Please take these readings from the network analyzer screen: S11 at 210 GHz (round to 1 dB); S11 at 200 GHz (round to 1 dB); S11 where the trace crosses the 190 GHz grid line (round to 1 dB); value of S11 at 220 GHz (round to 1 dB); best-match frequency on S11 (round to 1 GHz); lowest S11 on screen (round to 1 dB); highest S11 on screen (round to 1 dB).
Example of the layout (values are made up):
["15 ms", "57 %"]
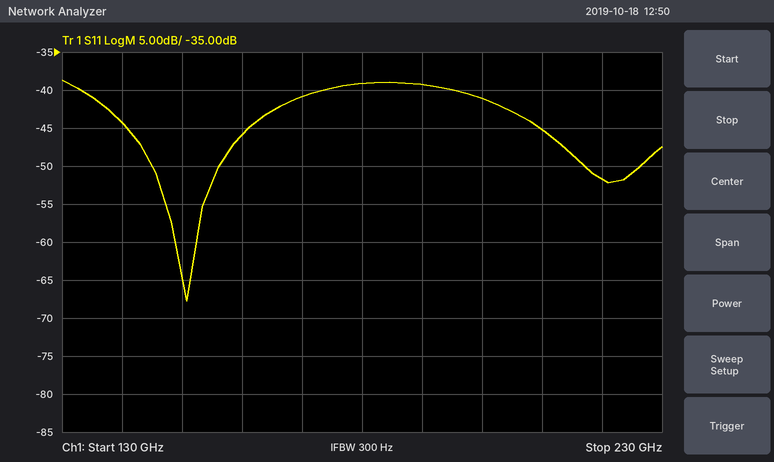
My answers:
["-45 dB", "-41 dB", "-39 dB", "-52 dB", "151 GHz", "-68 dB", "-39 dB"]
